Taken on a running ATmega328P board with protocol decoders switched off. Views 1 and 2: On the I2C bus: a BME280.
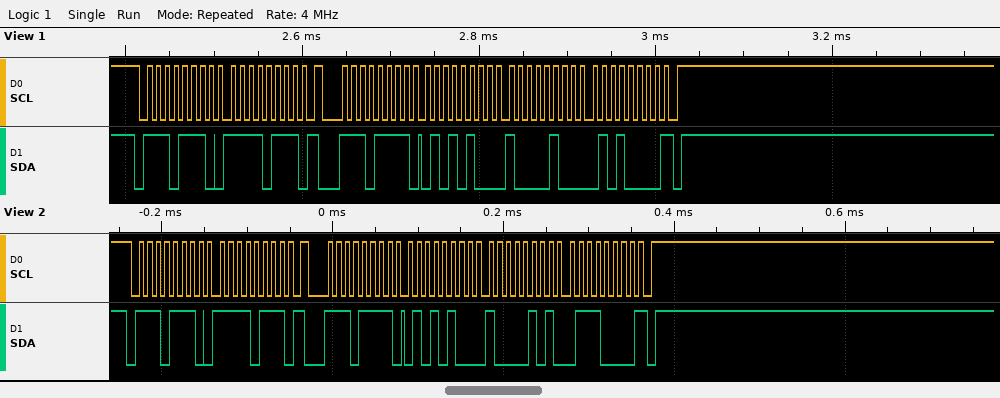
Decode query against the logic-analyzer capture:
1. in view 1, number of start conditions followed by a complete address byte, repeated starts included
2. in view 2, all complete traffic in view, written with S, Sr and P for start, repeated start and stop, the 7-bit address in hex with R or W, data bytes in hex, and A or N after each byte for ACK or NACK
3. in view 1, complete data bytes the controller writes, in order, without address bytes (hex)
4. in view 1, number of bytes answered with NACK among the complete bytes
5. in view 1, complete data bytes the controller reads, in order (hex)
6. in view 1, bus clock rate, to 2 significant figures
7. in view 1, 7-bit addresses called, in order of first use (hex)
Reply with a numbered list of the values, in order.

1. 2
2. S 77W A F7 A Sr 77R A 54 A 85 A 70 N P
3. F7
4. 1
5. 54 84 50
6. 100 kHz
7. 0x77
